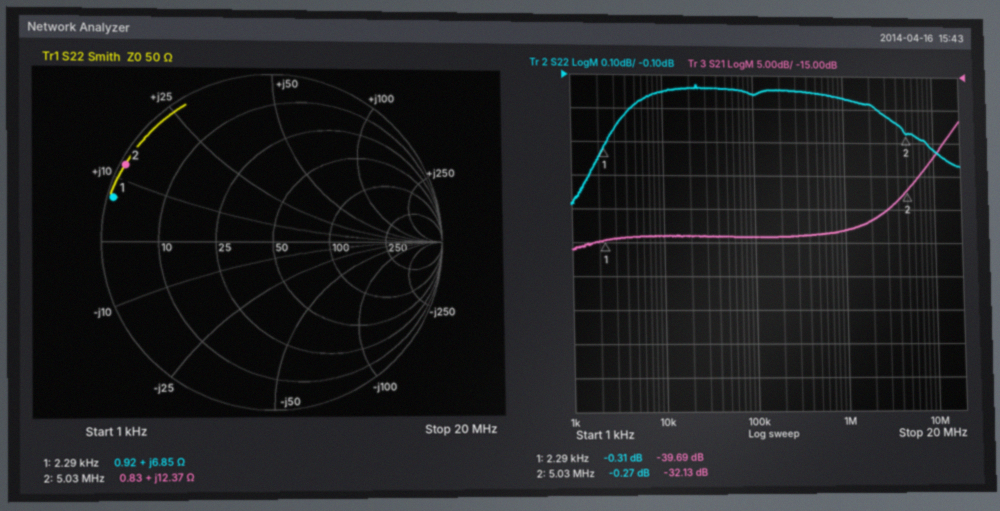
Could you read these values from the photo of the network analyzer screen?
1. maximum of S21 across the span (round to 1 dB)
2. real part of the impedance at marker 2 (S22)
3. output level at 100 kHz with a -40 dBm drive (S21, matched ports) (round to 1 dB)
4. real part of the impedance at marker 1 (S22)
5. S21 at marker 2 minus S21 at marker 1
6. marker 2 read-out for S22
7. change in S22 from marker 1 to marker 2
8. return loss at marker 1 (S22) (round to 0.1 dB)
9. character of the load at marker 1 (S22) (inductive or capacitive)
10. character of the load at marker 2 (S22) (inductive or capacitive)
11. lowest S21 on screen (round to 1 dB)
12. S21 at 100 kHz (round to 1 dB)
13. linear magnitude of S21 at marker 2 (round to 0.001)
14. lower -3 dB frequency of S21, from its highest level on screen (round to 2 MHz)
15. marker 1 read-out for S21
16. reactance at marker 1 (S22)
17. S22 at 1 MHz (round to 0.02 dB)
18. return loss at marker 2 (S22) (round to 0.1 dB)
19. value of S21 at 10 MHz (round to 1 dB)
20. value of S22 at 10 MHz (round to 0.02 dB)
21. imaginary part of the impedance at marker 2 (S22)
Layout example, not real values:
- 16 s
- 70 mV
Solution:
- -22 dB
- 0.83 Ω
- -79 dBm
- 0.92 Ω
- 7.56 dB
- -0.27 dB
- 0.04 dB
- 0.3 dB
- inductive
- inductive
- -41 dB
- -39 dB
- 0.025
- 14 MHz
- -39.69 dB
- +6.85 Ω
- -0.16 dB
- 0.3 dB
- -27 dB
- -0.32 dB
- +12.37 Ω
